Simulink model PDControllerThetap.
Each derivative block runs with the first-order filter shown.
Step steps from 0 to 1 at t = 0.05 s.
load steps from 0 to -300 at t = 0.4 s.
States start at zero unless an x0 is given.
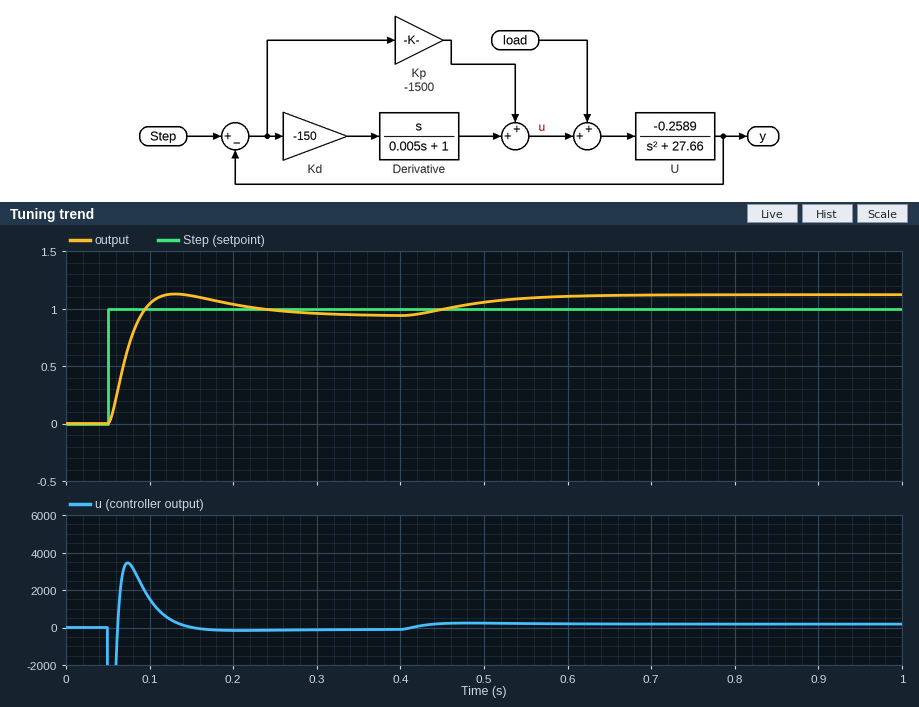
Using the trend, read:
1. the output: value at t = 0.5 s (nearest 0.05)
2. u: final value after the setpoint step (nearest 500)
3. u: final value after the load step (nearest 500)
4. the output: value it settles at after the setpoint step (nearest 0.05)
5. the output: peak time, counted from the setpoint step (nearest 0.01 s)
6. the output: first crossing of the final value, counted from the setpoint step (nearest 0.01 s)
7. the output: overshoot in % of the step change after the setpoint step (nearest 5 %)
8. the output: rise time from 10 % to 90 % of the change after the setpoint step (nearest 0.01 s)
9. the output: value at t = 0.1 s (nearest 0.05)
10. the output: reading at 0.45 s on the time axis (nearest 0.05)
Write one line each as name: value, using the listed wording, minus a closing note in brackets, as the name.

the output: value at t = 0.5 s: 1.05
u: final value after the setpoint step: 0
u: final value after the load step: 0
the output: value it settles at after the setpoint step: 0.95
the output: peak time, counted from the setpoint step: 0.08 s
the output: first crossing of the final value, counted from the setpoint step: 0.04 s
the output: overshoot in % of the step change after the setpoint step: 20 %
the output: rise time from 10 % to 90 % of the change after the setpoint step: 0.03 s
the output: value at t = 0.1 s: 1.05
the output: reading at 0.45 s on the time axis: 1.00
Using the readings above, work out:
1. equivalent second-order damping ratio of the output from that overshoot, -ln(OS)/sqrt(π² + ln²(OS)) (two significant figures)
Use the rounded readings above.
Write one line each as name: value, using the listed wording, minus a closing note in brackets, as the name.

equivalent second-order damping ratio of the output from that overshoot, -ln(OS)/sqrt(π² + ln²(OS)): 0.46
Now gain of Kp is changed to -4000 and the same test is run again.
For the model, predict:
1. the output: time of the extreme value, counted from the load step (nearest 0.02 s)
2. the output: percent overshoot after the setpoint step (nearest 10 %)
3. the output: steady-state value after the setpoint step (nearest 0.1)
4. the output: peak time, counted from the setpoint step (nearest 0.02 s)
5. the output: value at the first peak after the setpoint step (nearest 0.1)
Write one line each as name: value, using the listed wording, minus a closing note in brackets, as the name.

the output: time of the extreme value, counted from the load step: 0.12 s
the output: percent overshoot after the setpoint step: 30 %
the output: steady-state value after the setpoint step: 1.0
the output: peak time, counted from the setpoint step: 0.06 s
the output: value at the first peak after the setpoint step: 1.3
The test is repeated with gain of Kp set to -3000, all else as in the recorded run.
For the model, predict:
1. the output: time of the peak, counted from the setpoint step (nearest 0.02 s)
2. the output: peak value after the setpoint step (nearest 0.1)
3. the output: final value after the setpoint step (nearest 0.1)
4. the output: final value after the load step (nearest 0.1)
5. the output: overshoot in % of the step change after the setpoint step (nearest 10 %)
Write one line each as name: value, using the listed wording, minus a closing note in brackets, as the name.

the output: time of the peak, counted from the setpoint step: 0.06 s
the output: peak value after the setpoint step: 1.2
the output: final value after the setpoint step: 1.0
the output: final value after the load step: 1.1
the output: overshoot in % of the step change after the setpoint step: 30 %
